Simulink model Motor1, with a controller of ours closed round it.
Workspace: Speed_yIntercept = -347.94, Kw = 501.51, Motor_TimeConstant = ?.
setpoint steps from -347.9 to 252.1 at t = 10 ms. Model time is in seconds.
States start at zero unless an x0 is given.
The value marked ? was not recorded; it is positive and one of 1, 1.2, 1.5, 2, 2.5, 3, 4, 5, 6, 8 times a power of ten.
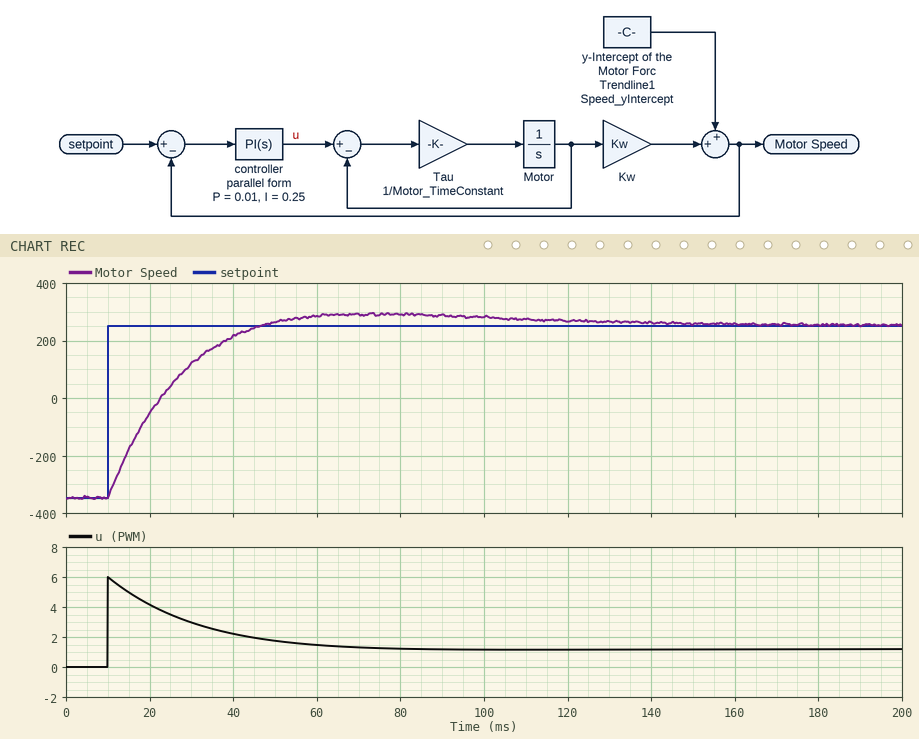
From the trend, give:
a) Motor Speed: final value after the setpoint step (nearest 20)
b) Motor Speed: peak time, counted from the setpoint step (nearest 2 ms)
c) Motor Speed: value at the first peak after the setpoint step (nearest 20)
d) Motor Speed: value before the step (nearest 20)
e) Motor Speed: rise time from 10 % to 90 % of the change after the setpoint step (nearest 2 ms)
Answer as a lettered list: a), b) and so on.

a) 260
b) 62 ms
c) 300
d) -340
e) 26 ms
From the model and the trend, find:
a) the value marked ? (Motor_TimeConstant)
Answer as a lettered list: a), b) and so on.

a) 0.08
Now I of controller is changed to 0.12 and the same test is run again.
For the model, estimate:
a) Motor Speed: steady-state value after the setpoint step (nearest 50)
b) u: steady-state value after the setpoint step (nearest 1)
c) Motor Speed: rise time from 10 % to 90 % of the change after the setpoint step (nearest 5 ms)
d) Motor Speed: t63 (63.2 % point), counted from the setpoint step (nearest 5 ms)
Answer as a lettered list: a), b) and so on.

a) 250
b) 1
c) 35 ms
d) 15 ms
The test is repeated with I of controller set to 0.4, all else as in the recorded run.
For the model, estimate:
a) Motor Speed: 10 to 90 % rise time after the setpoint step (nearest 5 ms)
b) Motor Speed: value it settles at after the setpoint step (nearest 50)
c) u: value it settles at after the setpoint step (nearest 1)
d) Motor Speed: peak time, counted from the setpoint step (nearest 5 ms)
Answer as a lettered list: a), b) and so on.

a) 20 ms
b) 250
c) 1
d) 50 ms
